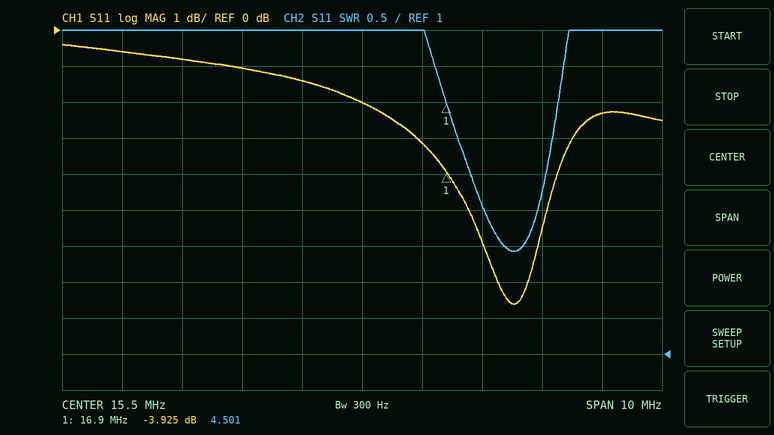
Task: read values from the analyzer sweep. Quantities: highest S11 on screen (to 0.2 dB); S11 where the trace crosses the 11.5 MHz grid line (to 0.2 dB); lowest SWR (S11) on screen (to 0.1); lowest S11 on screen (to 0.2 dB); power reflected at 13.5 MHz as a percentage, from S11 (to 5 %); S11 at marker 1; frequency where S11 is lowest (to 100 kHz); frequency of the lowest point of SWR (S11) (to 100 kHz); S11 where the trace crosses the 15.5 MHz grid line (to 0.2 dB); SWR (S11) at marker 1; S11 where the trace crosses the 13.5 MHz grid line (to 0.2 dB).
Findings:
-0.4 dB
-0.6 dB
2.4
-7.6 dB
80 %
-3.925 dB
18.0 MHz
18.0 MHz
-2.0 dB
4.501
-1.0 dB
